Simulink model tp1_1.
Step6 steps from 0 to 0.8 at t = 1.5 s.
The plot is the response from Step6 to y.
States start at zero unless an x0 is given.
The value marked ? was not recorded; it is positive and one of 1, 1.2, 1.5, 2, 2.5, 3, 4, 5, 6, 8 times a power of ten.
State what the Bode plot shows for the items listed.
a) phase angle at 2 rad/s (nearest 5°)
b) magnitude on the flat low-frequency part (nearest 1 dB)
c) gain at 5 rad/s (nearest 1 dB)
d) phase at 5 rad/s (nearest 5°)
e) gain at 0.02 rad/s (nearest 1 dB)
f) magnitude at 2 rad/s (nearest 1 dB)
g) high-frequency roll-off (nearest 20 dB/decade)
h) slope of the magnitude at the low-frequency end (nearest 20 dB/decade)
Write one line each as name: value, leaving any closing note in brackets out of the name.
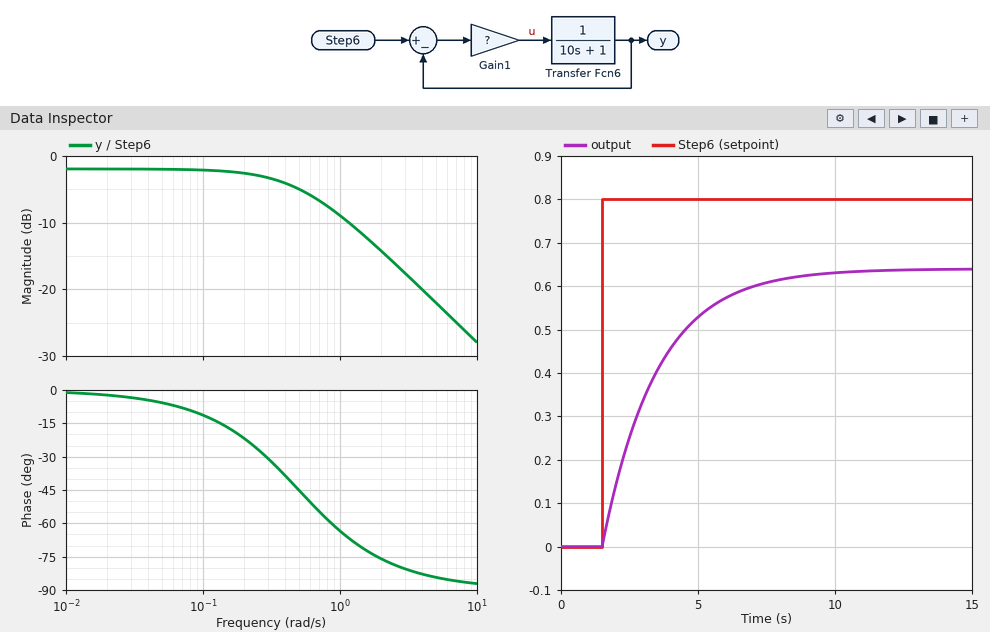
phase angle at 2 rad/s: -75°
magnitude on the flat low-frequency part: -2 dB
gain at 5 rad/s: -22 dB
phase at 5 rad/s: -85°
gain at 0.02 rad/s: -2 dB
magnitude at 2 rad/s: -14 dB
high-frequency roll-off: -20 dB/decade
slope of the magnitude at the low-frequency end: 0 dB/decade
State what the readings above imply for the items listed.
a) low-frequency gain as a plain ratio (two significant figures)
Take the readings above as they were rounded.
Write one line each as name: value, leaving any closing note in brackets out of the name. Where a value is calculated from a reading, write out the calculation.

low-frequency gain as a plain ratio: 10^(-2 / 20) = 0.79
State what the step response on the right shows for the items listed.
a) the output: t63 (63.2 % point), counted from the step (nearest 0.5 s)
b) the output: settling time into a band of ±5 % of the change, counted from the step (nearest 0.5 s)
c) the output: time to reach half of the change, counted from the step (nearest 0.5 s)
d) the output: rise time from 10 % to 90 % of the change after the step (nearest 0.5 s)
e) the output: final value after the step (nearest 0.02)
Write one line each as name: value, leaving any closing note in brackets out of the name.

the output: t63 (63.2 % point), counted from the step: 2.0 s
the output: settling time into a band of ±5 % of the change, counted from the step: 6.0 s
the output: time to reach half of the change, counted from the step: 1.5 s
the output: rise time from 10 % to 90 % of the change after the step: 4.5 s
the output: final value after the step: 0.64
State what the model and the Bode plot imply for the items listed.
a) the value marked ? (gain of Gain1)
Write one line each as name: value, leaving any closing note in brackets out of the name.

the value marked ?: 4
